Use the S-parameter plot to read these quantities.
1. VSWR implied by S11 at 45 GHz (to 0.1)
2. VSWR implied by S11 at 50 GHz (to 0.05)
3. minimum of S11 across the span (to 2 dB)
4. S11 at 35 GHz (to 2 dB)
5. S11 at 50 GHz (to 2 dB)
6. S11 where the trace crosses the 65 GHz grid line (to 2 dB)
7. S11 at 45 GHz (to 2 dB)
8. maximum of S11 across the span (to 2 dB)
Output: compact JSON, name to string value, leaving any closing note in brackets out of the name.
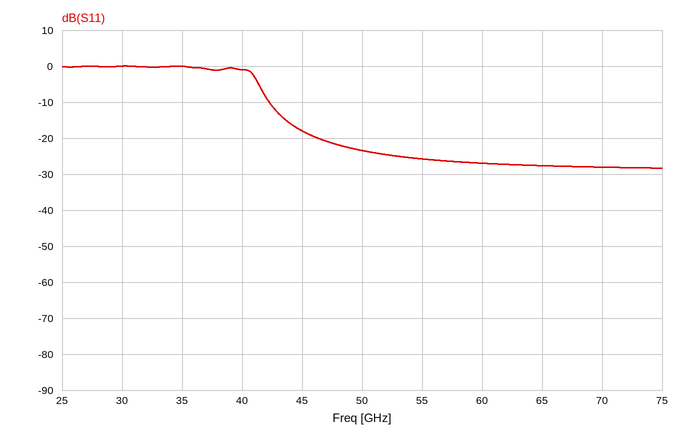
{"VSWR implied by S11 at 45 GHz": "1.3", "VSWR implied by S11 at 50 GHz": "1.15", "minimum of S11 across the span": "-28 dB", "S11 at 35 GHz": "0 dB", "S11 at 50 GHz": "-24 dB", "S11 where the trace crosses the 65 GHz grid line": "-28 dB", "S11 at 45 GHz": "-18 dB", "maximum of S11 across the span": "0 dB"}
